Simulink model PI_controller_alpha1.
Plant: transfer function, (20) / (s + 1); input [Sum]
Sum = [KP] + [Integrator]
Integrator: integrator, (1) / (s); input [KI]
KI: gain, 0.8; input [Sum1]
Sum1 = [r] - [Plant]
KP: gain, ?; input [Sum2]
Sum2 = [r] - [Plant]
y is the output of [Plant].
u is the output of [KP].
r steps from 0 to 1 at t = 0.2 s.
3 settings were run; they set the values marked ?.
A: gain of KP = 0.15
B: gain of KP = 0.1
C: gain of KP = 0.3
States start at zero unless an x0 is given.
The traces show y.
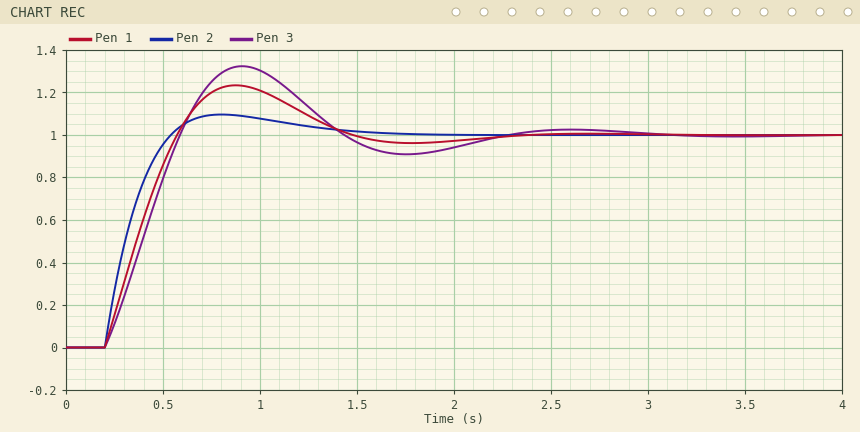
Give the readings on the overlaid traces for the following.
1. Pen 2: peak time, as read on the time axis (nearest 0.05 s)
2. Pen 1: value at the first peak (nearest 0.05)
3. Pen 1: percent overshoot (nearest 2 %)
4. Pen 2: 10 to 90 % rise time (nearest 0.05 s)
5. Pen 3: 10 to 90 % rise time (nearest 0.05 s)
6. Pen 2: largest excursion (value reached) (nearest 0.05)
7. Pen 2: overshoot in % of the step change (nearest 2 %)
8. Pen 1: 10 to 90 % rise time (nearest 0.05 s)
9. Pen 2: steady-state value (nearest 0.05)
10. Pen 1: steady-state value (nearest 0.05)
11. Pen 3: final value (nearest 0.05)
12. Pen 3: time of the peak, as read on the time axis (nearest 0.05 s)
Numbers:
0.80 s
1.25
24 %
0.25 s
0.30 s
1.10
10 %
0.30 s
1.00
1.00
1.00
0.90 s
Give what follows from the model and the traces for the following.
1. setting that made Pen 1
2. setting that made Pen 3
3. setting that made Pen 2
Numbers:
A
B
C
